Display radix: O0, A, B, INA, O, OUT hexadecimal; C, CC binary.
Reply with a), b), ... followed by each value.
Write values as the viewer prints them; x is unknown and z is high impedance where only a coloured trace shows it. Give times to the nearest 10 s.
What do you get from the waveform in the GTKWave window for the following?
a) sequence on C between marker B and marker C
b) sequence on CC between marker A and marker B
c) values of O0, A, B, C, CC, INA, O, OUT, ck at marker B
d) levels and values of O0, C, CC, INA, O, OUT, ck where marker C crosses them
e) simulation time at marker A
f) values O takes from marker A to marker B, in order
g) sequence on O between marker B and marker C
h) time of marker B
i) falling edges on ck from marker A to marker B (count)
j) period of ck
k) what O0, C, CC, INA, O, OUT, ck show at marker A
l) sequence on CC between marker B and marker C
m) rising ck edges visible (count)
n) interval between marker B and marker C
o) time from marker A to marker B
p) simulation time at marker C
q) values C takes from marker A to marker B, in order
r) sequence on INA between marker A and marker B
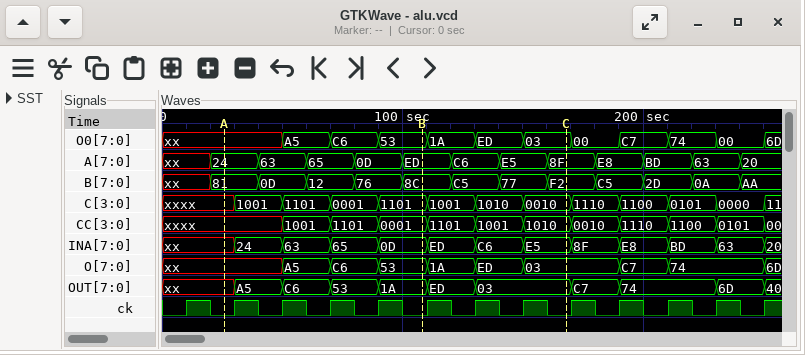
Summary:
a) 1101, 1001, 1010, 0010
b) xxxx, 1001, 1101, 0001
c) O0=53, A=ED, B=8C, C=1101, CC=0001, INA=0D, O=53, OUT=1A, ck=0
d) O0=03, C=0010, CC=1010, INA=E5, O=03, OUT=03, ck=0
e) 30 s
f) xx, A5, C6, 53
g) 53, 1A, ED, 03
h) 110 s
i) 4
j) 20 s
k) O0=xx, C=xxxx, CC=xxxx, INA=xx, O=xx, OUT=xx, ck=0
l) 0001, 1101, 1001, 1010
m) 13
n) 60 s
o) 80 s
p) 170 s
q) xxxx, 1001, 1101, 0001, 1101
r) xx, 24, 63, 65, 0D
